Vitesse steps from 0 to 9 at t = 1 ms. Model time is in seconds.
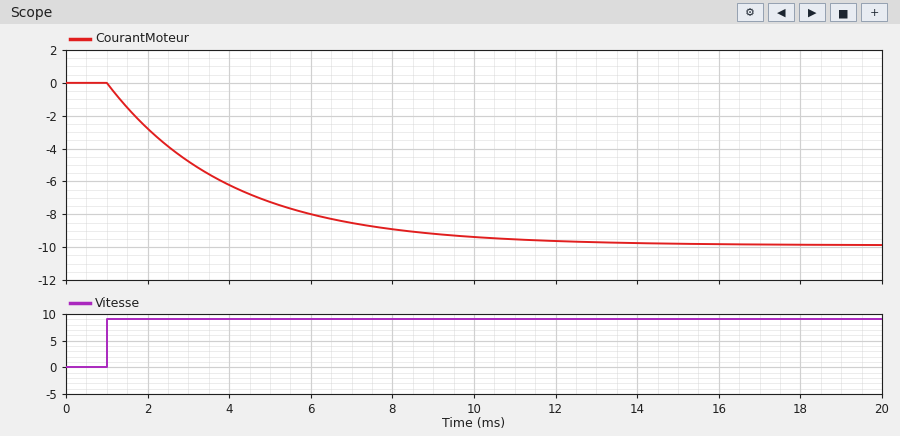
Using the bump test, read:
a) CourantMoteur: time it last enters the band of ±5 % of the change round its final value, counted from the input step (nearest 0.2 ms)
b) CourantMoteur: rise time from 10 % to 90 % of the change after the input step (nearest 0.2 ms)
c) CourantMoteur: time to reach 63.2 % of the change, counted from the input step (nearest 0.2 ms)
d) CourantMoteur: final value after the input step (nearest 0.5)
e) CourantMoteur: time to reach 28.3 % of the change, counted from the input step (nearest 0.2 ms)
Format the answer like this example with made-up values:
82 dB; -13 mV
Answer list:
9.0 ms; 6.6 ms; 3.0 ms; -10.0; 1.0 ms
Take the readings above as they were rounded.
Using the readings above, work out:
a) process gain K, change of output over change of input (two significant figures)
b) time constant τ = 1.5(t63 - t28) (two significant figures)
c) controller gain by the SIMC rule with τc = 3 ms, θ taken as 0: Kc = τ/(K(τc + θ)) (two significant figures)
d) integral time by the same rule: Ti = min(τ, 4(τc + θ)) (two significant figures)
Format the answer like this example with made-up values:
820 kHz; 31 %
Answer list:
-1.1; 3.0 ms; -0.91; 3.0 ms
